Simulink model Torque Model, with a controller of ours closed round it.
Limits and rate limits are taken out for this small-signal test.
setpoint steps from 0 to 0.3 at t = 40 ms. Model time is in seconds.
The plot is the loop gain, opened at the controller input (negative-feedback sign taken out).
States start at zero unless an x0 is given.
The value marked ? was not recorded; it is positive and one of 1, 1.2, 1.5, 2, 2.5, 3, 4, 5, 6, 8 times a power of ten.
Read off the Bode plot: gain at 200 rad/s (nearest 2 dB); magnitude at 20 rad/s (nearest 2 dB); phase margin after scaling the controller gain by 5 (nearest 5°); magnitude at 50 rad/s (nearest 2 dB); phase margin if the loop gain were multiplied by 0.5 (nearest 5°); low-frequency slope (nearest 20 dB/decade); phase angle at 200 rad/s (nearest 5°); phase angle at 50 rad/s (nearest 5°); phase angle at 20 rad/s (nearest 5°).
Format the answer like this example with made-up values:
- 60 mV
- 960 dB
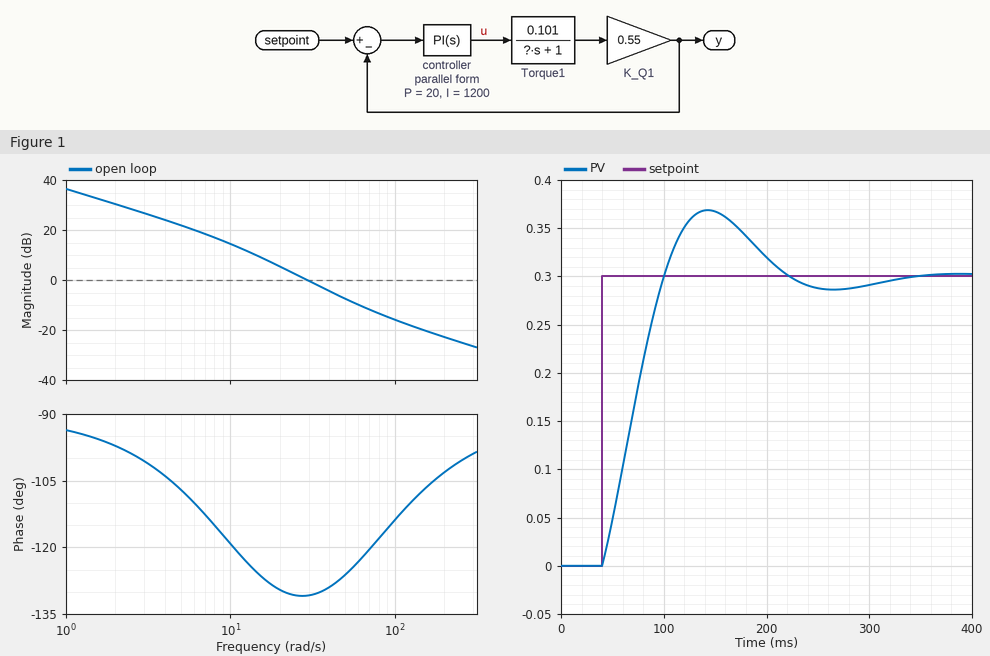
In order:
- -22 dB
- 6 dB
- 65°
- -8 dB
- 50°
- -20 dB/decade
- -105°
- -125°
- -130°
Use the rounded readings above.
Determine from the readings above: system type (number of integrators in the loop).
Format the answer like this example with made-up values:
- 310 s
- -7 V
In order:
- 1
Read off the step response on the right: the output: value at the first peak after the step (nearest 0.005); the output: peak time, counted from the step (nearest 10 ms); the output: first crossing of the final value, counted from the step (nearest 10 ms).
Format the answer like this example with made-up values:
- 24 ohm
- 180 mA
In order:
- 0.370
- 100 ms
- 60 ms
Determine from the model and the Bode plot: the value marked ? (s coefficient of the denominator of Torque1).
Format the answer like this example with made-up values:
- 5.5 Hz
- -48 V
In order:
- 0.08
